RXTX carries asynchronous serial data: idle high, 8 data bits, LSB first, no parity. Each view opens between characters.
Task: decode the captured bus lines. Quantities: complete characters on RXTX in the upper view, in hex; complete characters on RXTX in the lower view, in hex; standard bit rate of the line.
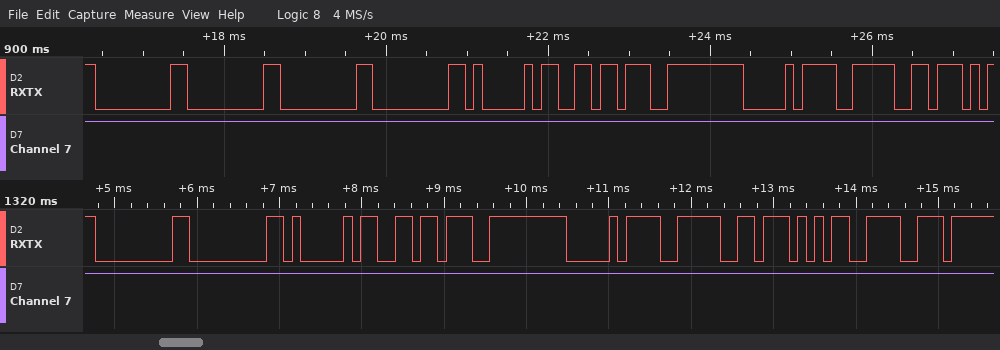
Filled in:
00, 00, 00, 00, 41, B6, FE, D0, 3E
00, 00, 41, B6, FE, D0, 3E, 57, 9E
9600 baud
